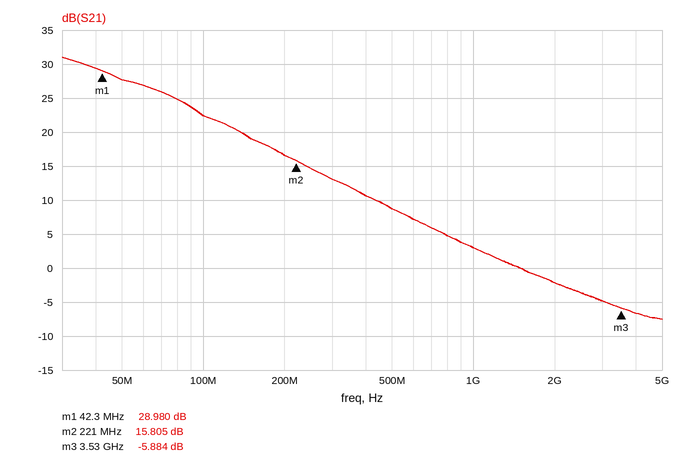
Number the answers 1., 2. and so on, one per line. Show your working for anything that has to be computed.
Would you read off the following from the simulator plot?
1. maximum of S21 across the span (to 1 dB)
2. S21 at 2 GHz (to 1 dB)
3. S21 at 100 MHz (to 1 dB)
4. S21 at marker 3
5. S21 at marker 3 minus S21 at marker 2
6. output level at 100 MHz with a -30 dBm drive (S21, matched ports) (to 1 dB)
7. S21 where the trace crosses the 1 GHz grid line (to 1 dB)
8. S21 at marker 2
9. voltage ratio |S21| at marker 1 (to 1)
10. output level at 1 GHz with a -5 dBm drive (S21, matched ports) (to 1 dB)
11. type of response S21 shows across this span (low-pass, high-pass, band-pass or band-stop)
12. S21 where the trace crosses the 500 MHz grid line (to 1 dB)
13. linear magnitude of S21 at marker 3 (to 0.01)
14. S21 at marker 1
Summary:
1. 31 dB
2. -2 dB
3. 22 dB
4. -5.884 dB
5. -5.884 − (15.805) = -21.689 dB
6. -30 dBm + (22 dB) = -8 dBm
7. 3 dB
8. 15.805 dB
9. 10^(28.98/20) ≈ 28
10. -5 dBm + (3 dB) = -2 dBm
11. low-pass
12. 9 dB
13. 10^(-5.884/20) ≈ 0.51
14. 28.980 dB
